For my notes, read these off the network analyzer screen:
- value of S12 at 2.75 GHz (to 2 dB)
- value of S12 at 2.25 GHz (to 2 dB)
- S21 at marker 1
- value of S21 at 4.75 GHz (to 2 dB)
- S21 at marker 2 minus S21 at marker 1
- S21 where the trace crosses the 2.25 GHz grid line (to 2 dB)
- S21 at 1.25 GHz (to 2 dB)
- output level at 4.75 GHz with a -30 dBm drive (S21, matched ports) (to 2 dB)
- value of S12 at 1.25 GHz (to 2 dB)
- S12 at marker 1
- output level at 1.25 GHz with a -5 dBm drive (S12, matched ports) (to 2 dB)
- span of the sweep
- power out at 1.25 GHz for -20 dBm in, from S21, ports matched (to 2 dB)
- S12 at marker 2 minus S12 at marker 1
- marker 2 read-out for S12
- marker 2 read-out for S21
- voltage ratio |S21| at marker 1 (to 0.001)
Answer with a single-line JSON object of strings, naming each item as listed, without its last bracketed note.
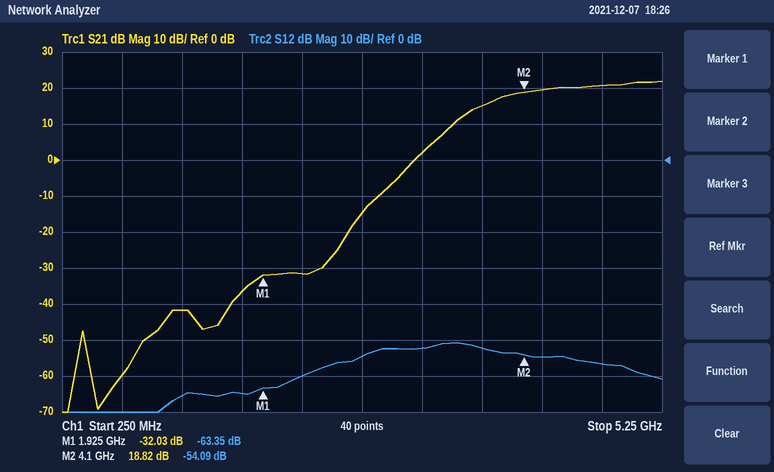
{"value of S12 at 2.75 GHz": "-54 dB", "value of S12 at 2.25 GHz": "-60 dB", "S21 at marker 1": "-32.03 dB", "value of S21 at 4.75 GHz": "20 dB", "S21 at marker 2 minus S21 at marker 1": "50.85 dB", "S21 where the trace crosses the 2.25 GHz grid line": "-32 dB", "S21 at 1.25 GHz": "-42 dB", "output level at 4.75 GHz with a -30 dBm drive (S21, matched ports)": "-10 dBm", "value of S12 at 1.25 GHz": "-66 dB", "S12 at marker 1": "-63.35 dB", "output level at 1.25 GHz with a -5 dBm drive (S12, matched ports)": "-70 dBm", "span of the sweep": "5 GHz", "power out at 1.25 GHz for -20 dBm in, from S21, ports matched": "-62 dBm", "S12 at marker 2 minus S12 at marker 1": "9.26 dB", "marker 2 read-out for S12": "-54.09 dB", "marker 2 read-out for S21": "18.82 dB", "voltage ratio |S21| at marker 1": "0.025"}
